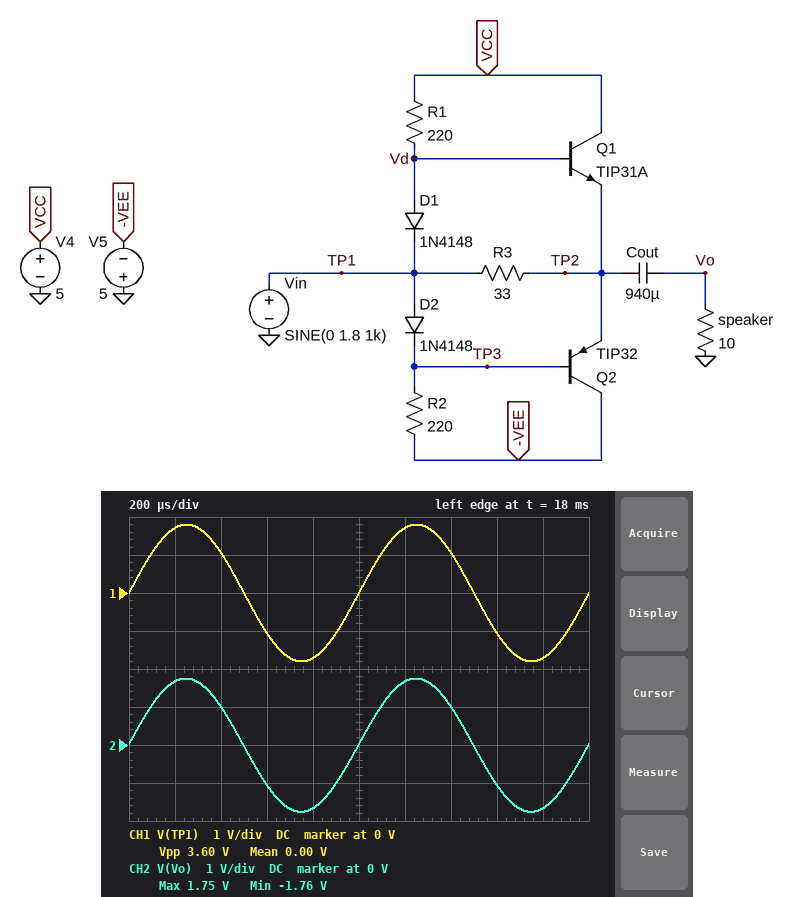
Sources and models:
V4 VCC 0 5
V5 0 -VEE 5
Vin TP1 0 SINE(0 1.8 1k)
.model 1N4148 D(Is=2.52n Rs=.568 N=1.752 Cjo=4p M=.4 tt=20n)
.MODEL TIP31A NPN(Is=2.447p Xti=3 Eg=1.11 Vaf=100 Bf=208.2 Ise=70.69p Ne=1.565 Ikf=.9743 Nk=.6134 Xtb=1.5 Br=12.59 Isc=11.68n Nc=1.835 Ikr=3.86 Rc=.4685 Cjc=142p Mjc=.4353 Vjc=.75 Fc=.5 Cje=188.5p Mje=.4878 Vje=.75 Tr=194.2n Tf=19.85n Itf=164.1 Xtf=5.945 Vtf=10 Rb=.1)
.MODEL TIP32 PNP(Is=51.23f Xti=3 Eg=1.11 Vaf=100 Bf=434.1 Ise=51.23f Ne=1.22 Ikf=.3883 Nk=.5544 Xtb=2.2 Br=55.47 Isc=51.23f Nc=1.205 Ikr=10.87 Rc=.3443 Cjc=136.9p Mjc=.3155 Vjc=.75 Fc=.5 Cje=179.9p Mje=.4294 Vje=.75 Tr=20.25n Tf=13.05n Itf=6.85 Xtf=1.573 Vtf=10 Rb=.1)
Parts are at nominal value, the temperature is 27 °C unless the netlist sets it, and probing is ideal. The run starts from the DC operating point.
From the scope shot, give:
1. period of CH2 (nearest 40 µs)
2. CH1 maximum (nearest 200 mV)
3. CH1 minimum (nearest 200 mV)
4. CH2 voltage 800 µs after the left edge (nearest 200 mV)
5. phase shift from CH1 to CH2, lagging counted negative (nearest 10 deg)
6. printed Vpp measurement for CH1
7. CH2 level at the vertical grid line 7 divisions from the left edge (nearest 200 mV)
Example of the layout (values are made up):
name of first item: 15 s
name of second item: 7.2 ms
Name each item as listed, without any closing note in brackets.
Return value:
period of CH2: 1.00 ms
CH1 maximum: 1.8 V
CH1 minimum: -1.8 V
CH2 voltage 800 µs after the left edge: -1.6 V
phase shift from CH1 to CH2, lagging counted negative: 0 deg
printed Vpp measurement for CH1: 3.60 V
CH2 level at the vertical grid line 7 divisions from the left edge: 1.0 V
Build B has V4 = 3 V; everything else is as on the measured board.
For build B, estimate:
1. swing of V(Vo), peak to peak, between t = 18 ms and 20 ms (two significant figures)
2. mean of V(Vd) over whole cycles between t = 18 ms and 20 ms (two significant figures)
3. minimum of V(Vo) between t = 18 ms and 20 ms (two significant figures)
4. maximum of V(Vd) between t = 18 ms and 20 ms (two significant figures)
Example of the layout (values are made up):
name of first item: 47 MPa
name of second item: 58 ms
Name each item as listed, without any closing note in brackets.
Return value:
swing of V(Vo), peak to peak, between t = 18 ms and 20 ms: 3.4 V
mean of V(Vd) over whole cycles between t = 18 ms and 20 ms: 670 mV
minimum of V(Vo) between t = 18 ms and 20 ms: -1.7 V
maximum of V(Vd) between t = 18 ms and 20 ms: 2.4 V
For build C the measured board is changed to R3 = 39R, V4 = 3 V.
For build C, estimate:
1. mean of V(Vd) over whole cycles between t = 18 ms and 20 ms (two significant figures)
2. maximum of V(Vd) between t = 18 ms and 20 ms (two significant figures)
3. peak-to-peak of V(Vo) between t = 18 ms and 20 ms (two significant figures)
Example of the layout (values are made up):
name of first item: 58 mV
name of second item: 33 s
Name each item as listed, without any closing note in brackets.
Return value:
mean of V(Vd) over whole cycles between t = 18 ms and 20 ms: 670 mV
maximum of V(Vd) between t = 18 ms and 20 ms: 2.4 V
peak-to-peak of V(Vo) between t = 18 ms and 20 ms: 3.4 V
